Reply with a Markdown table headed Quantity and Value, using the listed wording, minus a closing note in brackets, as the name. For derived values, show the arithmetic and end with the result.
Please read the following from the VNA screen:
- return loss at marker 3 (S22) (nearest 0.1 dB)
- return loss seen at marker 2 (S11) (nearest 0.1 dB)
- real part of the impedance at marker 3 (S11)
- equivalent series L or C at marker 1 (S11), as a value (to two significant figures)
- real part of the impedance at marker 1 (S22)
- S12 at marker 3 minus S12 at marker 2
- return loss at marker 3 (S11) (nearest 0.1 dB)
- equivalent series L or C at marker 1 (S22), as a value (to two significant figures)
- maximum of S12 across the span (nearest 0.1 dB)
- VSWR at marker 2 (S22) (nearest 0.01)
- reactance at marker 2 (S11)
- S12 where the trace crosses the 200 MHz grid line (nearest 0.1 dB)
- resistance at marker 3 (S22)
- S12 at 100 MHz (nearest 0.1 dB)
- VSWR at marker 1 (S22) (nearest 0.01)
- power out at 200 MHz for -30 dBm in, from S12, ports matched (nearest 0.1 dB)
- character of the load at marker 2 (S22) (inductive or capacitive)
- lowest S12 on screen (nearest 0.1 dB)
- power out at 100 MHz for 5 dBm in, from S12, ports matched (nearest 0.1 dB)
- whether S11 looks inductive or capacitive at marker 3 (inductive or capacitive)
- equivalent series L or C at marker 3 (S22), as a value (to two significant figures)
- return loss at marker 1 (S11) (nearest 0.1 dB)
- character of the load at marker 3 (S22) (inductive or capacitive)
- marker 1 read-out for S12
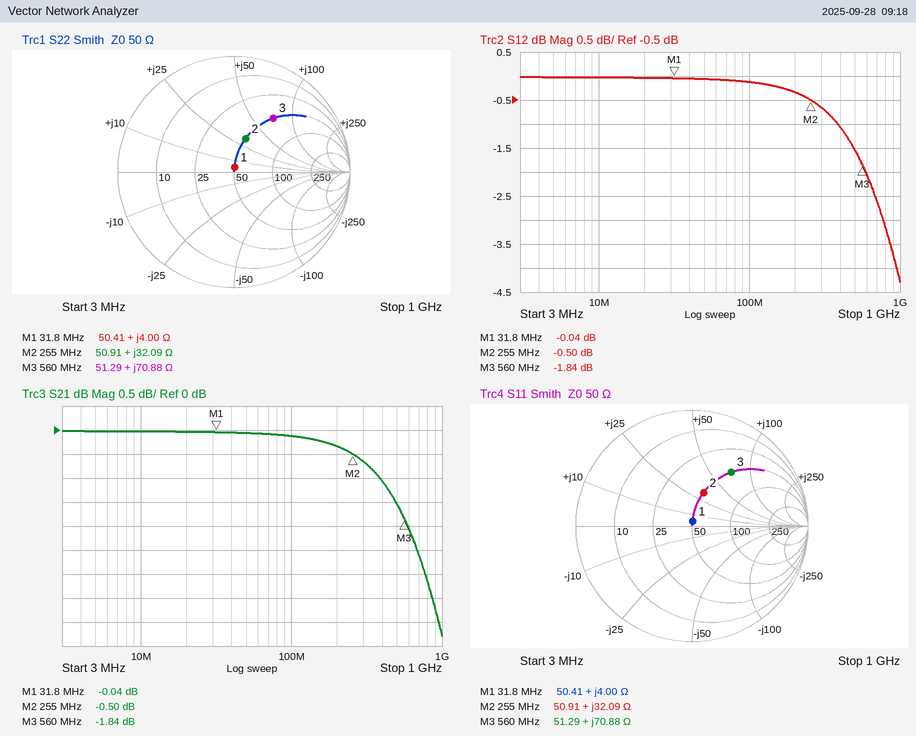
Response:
| Quantity | Value |
|---|---|
| return loss at marker 3 (S22) | 4.8 dB |
| return loss seen at marker 2 (S11) | 10.4 dB |
| real part of the impedance at marker 3 | 51.29 Ω |
| equivalent series L or C at marker 1 (S11), as a value | L = 4 Ω/(2π × 31.8 MHz) ≈ 20 nH |
| real part of the impedance at marker 1 | 50.41 Ω |
| S12 at marker 3 minus S12 at marker 2 | -1.84 − (-0.5) = -1.34 dB |
| return loss at marker 3 (S11) | 4.8 dB |
| equivalent series L or C at marker 1 (S22), as a value | L = 4 Ω/(2π × 31.8 MHz) ≈ 20 nH |
| maximum of S12 across the span | 0.0 dB |
| VSWR at marker 2 (S22) | 1.87 |
| reactance at marker 2 | +32.09 Ω |
| S12 where the trace crosses the 200 MHz grid line | -0.3 dB |
| resistance at marker 3 | 51.29 Ω |
| S12 at 100 MHz | -0.1 dB |
| VSWR at marker 1 (S22) | 1.08 |
| power out at 200 MHz for -30 dBm in, from S12, ports matched | -30 dBm + (-0.3 dB) = -30.3 dBm |
| character of the load at marker 2 (S22) | inductive |
| lowest S12 on screen | -4.3 dB |
| power out at 100 MHz for 5 dBm in, from S12, ports matched | 5 dBm + (-0.1 dB) = 4.9 dBm |
| whether S11 looks inductive or capacitive at marker 3 | inductive |
| equivalent series L or C at marker 3 (S22), as a value | L = 70.88 Ω/(2π × 560 MHz) ≈ 20 nH |
| return loss at marker 1 (S11) | 28.0 dB |
| character of the load at marker 3 (S22) | inductive |
| marker 1 read-out for S12 | -0.04 dB |
